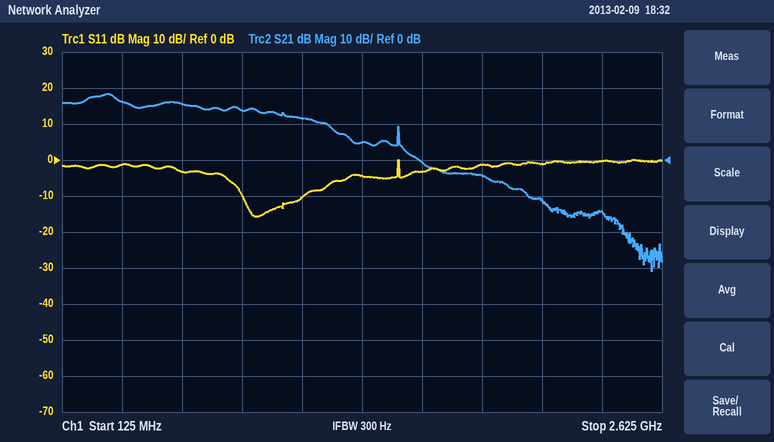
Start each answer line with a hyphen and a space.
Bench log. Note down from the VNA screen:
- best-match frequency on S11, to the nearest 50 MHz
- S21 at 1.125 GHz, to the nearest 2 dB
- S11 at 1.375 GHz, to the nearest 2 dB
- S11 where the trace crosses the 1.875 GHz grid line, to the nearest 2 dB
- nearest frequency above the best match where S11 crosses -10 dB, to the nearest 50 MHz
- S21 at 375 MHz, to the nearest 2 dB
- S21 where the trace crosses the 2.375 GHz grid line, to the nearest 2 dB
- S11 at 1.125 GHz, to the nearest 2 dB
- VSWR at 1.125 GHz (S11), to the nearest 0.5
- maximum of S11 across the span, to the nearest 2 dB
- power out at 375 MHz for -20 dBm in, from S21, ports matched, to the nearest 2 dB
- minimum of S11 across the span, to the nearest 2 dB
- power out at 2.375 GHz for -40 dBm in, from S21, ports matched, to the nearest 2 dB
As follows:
- 950 MHz
- 12 dB
- -4 dB
- -2 dB
- 1.15 GHz
- 16 dB
- -14 dB
- -10 dB
- 2.0
- 0 dB
- -4 dBm
- -16 dB
- -54 dBm
